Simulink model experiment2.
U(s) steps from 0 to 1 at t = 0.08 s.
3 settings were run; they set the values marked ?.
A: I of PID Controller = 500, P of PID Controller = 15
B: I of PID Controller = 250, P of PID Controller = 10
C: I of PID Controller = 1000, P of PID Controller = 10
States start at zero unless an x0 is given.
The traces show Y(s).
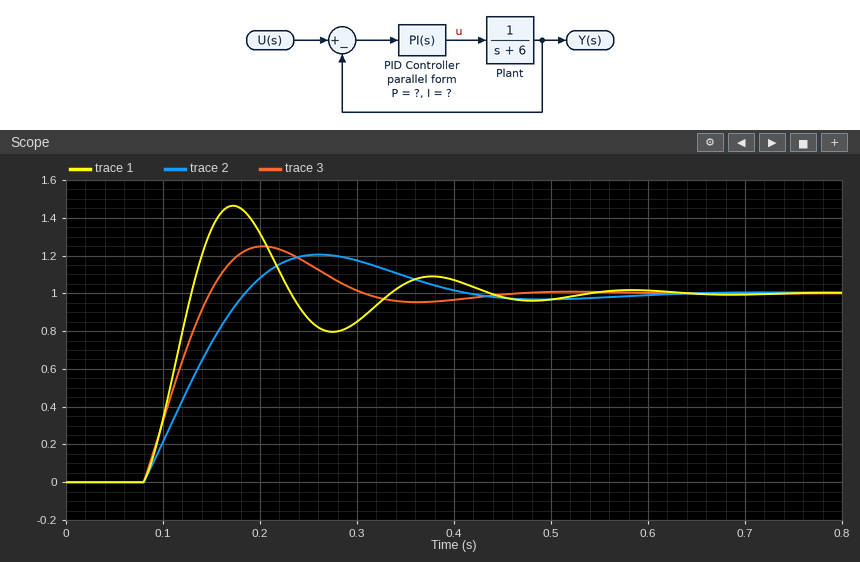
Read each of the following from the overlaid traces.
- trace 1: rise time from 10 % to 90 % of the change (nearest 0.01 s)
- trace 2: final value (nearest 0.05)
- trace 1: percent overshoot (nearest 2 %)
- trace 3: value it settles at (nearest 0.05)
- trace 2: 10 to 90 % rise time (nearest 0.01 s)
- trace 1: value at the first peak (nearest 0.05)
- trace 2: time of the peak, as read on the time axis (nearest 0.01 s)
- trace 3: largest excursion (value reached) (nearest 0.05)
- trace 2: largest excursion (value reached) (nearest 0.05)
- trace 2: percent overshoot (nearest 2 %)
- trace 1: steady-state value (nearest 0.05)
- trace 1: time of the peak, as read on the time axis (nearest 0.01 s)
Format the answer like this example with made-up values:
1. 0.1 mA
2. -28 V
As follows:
1. 0.04 s
2. 1.00
3. 46 %
4. 1.00
5. 0.08 s
6. 1.45
7. 0.26 s
8. 1.25
9. 1.20
10. 20 %
11. 1.00
12. 0.17 s
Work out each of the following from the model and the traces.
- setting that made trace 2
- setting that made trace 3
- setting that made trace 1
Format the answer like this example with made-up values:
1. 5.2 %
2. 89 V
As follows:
1. B
2. A
3. C
